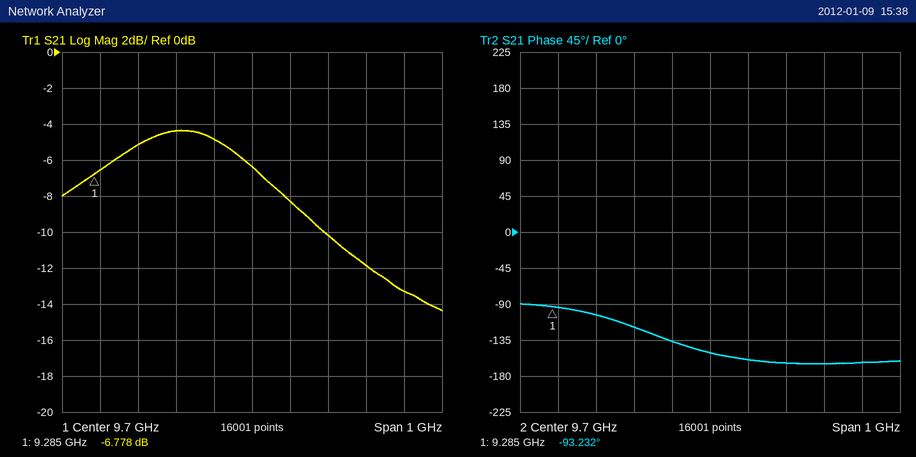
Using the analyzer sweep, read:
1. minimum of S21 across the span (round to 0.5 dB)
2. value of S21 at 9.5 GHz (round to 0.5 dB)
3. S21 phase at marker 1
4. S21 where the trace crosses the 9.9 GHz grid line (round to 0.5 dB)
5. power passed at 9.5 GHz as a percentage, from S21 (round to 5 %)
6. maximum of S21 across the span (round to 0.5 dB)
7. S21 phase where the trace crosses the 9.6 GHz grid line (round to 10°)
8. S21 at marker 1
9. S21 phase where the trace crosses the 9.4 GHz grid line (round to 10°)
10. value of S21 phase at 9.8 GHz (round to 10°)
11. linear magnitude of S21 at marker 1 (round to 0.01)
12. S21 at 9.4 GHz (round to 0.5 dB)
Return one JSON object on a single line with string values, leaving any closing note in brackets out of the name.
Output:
{"minimum of S21 across the span": "-14.5 dB", "value of S21 at 9.5 GHz": "-4.5 dB", "S21 phase at marker 1": "-93.232°", "S21 where the trace crosses the 9.9 GHz grid line": "-10.0 dB", "power passed at 9.5 GHz as a percentage, from S21": "35 %", "maximum of S21 across the span": "-4.5 dB", "S21 phase where the trace crosses the 9.6 GHz grid line": "-140°", "S21 at marker 1": "-6.778 dB", "S21 phase where the trace crosses the 9.4 GHz grid line": "-100°", "value of S21 phase at 9.8 GHz": "-160°", "linear magnitude of S21 at marker 1": "0.46", "S21 at 9.4 GHz": "-5.0 dB"}
